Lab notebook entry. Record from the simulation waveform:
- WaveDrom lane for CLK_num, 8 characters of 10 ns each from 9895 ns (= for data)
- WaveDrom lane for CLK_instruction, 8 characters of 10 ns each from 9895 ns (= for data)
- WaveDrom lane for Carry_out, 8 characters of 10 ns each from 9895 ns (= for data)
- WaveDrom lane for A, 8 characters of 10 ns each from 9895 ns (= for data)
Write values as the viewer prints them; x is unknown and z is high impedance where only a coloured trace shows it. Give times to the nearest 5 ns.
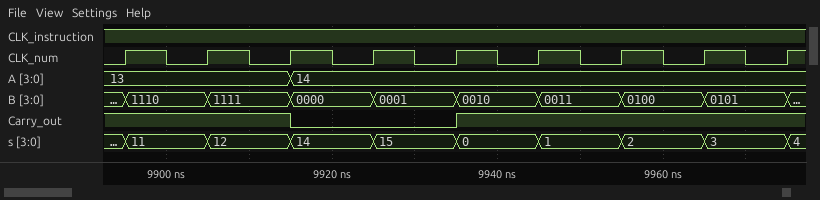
{name: 'CLK_num', wave: 'p.......'}
{name: 'CLK_instruction', wave: '1.......'}
{name: 'Carry_out', wave: '1.0.1...'}
{name: 'A', wave: '=.=.....', data: '13 14'}
